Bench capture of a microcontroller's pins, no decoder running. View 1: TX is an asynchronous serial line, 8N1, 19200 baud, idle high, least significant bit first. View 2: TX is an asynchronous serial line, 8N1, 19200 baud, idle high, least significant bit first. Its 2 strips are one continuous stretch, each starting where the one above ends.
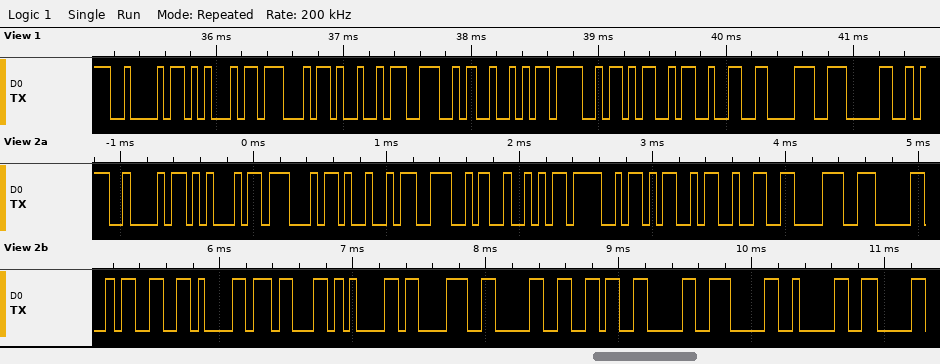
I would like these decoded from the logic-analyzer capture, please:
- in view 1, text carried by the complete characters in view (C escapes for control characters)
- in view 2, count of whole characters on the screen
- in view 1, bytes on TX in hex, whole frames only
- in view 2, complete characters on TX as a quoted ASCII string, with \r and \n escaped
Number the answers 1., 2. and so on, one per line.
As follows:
1. "BEGINROM280"
2. 21
3. 42 45 47 49 4E 52 4F 4D 32 38 30
4. "BEGINROM2803aca806000"
